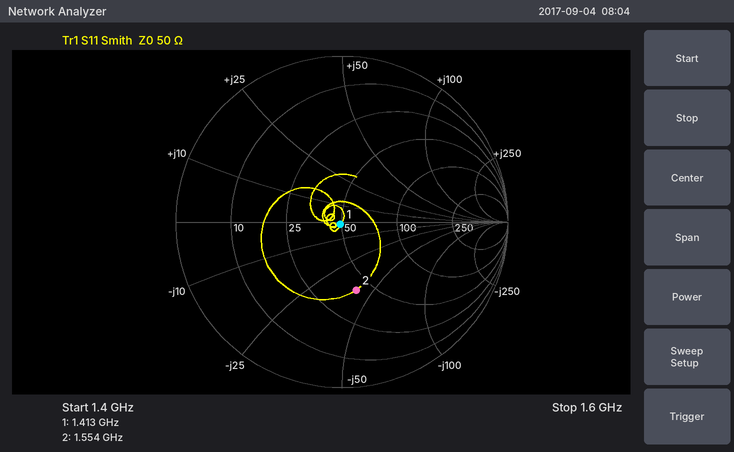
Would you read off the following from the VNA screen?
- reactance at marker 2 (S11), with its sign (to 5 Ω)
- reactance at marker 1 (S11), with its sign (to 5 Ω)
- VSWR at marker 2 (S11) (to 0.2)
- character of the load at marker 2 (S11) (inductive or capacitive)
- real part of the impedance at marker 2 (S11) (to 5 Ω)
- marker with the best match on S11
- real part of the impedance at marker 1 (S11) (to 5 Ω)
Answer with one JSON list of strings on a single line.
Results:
["-40 Ω", "0 Ω", "2.4", "capacitive", "40 Ω", "marker 1", "50 Ω"]
